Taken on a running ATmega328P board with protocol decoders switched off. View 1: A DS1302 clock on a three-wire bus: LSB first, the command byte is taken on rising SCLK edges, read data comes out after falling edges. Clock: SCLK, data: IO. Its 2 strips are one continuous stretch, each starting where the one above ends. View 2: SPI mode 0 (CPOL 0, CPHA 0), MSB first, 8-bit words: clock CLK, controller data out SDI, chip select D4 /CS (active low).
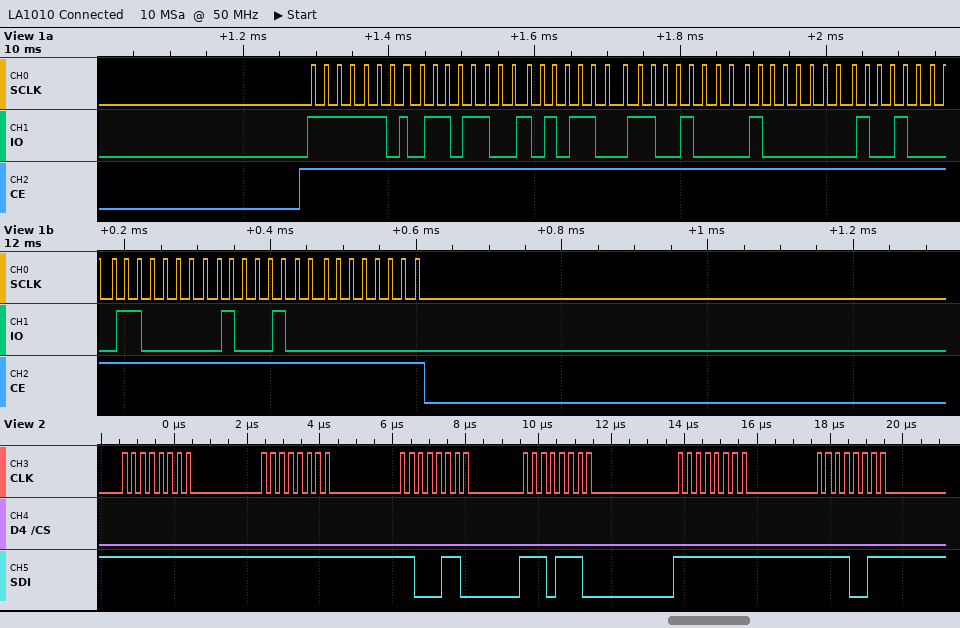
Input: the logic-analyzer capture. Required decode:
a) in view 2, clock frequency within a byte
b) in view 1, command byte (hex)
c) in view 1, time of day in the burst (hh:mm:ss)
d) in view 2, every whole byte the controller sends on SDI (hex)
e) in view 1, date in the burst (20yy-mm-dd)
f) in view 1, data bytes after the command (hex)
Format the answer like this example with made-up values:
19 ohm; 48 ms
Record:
4 MHz; 0xBF; 13:35:36; 0xFF 0xFF 0xC6 0xEE 0xFF 0xF3; 2022-12-02; 36 35 13 02 12 06 22 00
